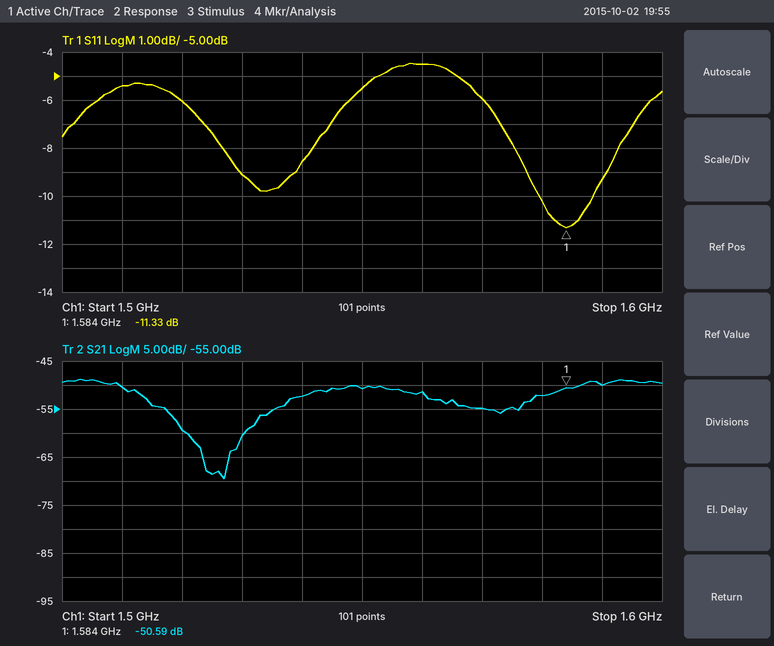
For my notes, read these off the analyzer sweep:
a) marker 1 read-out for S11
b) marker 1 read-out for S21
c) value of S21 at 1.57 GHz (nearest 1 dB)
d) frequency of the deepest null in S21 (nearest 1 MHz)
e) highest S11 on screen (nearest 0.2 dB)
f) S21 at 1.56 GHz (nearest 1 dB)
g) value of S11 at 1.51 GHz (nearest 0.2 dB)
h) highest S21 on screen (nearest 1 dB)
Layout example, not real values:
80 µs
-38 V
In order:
-11.33 dB
-50.59 dB
-55 dB
1.527 GHz
-4.4 dB
-51 dB
-5.4 dB
-49 dB
